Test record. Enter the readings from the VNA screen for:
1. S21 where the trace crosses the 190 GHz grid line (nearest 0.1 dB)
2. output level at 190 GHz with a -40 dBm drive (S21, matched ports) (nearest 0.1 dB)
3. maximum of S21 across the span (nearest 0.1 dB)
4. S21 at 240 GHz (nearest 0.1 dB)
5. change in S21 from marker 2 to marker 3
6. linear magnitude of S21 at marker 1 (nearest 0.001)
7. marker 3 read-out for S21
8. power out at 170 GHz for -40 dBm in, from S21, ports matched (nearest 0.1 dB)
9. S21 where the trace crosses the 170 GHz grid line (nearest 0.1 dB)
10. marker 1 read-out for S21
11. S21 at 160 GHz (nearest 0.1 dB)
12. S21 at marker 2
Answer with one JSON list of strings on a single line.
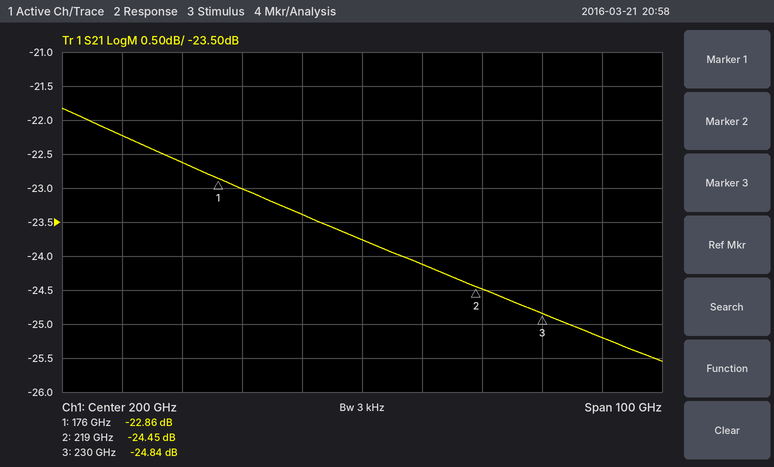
["-23.4 dB", "-63.4 dBm", "-21.8 dB", "-25.2 dB", "-0.39 dB", "0.072", "-24.84 dB", "-62.6 dBm", "-22.6 dB", "-22.86 dB", "-22.2 dB", "-24.45 dB"]
